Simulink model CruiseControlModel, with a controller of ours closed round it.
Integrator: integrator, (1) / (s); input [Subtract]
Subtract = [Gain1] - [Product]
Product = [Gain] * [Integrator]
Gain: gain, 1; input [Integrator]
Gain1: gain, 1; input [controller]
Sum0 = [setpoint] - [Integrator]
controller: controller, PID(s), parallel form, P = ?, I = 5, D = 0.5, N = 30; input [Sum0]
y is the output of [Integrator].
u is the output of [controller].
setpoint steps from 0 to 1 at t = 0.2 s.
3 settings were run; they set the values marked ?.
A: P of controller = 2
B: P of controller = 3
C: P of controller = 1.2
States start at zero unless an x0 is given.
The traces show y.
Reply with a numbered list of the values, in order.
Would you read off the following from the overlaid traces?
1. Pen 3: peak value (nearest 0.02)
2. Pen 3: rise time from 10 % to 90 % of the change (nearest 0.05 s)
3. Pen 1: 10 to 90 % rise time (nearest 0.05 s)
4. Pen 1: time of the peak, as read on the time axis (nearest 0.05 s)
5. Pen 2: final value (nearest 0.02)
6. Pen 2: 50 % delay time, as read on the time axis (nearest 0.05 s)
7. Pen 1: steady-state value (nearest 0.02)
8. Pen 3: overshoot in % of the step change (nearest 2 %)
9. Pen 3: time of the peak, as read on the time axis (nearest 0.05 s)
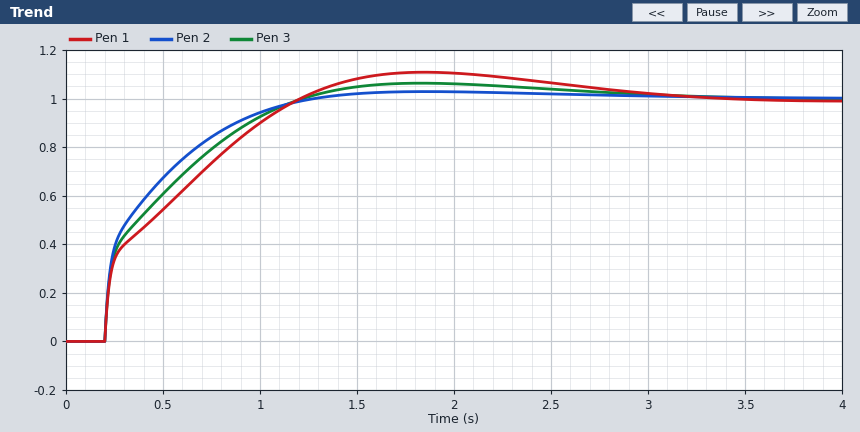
1. 1.06
2. 0.75 s
3. 0.80 s
4. 1.85 s
5. 1.00
6. 0.30 s
7. 1.00
8. 6 %
9. 1.85 s
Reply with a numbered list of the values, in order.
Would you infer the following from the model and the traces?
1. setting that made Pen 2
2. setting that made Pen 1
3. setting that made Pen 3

1. B
2. C
3. A
